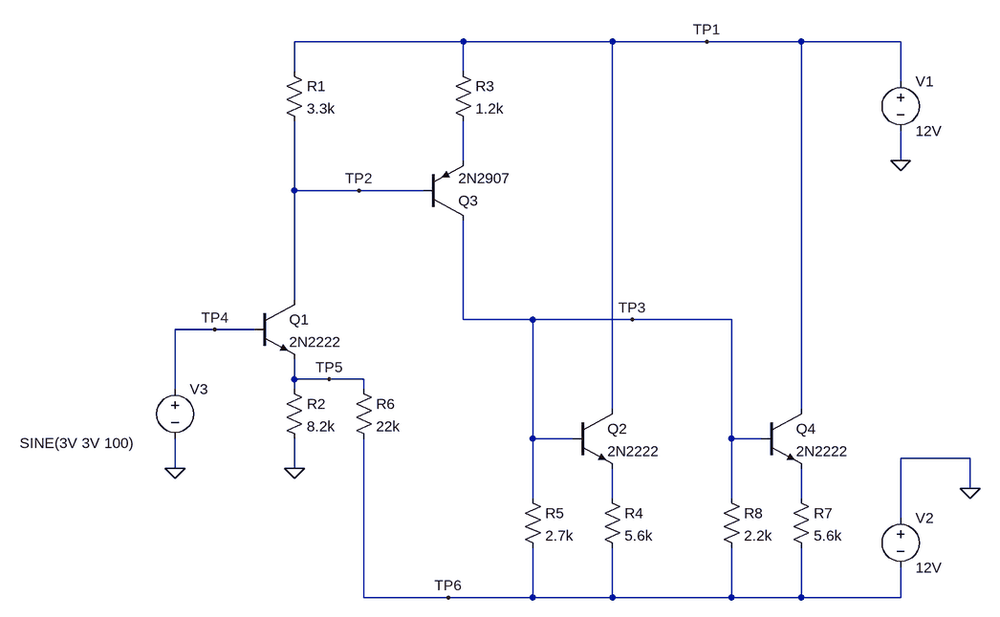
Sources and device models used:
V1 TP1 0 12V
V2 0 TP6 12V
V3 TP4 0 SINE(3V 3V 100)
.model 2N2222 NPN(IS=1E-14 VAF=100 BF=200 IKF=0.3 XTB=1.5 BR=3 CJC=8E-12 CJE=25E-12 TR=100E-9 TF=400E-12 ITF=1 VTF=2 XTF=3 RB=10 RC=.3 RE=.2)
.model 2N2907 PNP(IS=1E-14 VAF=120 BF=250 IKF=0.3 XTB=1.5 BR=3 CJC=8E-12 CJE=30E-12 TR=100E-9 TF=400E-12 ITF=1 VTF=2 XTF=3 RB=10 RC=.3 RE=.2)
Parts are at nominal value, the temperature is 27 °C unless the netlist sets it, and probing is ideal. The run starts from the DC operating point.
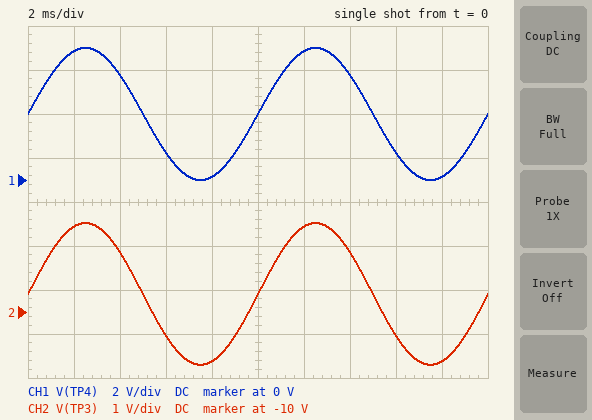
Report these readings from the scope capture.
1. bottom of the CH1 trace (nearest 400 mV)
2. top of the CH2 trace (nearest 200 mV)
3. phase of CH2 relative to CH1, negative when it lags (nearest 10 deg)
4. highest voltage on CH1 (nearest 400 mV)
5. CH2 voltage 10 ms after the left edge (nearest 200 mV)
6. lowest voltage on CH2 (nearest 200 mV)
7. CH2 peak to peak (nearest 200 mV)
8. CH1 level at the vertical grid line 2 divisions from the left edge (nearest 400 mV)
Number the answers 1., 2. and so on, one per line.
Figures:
1. 0 V
2. -8.0 V
3. 0 deg
4. 6.0 V
5. -9.6 V
6. -11.2 V
7. 3.2 V
8. 4.8 V
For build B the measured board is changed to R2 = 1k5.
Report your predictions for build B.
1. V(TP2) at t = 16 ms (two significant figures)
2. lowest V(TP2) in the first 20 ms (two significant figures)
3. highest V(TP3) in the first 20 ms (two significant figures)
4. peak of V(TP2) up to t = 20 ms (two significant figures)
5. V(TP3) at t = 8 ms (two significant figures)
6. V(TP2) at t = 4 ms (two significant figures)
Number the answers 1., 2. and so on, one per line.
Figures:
1. 8.9 V
2. 3.2 V
3. -3.8 V
4. 12 V
5. -12 V
6. 4.1 V
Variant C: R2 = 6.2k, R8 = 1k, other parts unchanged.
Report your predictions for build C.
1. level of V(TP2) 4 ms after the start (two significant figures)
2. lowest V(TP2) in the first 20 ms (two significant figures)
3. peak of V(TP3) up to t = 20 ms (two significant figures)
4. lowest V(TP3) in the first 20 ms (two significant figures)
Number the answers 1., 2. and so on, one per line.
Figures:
1. 7.5 V
2. 6.6 V
3. -9.2 V
4. -12 V
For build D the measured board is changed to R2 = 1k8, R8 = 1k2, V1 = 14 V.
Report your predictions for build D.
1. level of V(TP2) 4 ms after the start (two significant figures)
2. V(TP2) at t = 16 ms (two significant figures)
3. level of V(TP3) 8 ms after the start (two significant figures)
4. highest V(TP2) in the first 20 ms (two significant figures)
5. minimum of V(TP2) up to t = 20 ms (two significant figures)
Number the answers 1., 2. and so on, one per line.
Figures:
1. 4.3 V
2. 11 V
3. -12 V
4. 13 V
5. 4.2 V
